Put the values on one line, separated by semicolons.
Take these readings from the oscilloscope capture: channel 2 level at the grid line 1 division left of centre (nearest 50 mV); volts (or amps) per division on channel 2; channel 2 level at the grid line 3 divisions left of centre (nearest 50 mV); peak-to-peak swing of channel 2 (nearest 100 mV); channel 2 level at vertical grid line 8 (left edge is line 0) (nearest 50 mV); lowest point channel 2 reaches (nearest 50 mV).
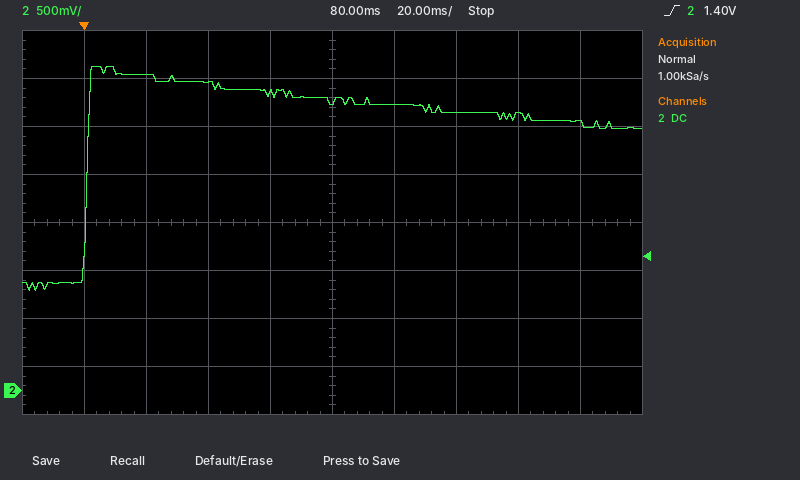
3.10 V; 500 mV; 3.30 V; 2.30 V; 2.90 V; 1.05 V
